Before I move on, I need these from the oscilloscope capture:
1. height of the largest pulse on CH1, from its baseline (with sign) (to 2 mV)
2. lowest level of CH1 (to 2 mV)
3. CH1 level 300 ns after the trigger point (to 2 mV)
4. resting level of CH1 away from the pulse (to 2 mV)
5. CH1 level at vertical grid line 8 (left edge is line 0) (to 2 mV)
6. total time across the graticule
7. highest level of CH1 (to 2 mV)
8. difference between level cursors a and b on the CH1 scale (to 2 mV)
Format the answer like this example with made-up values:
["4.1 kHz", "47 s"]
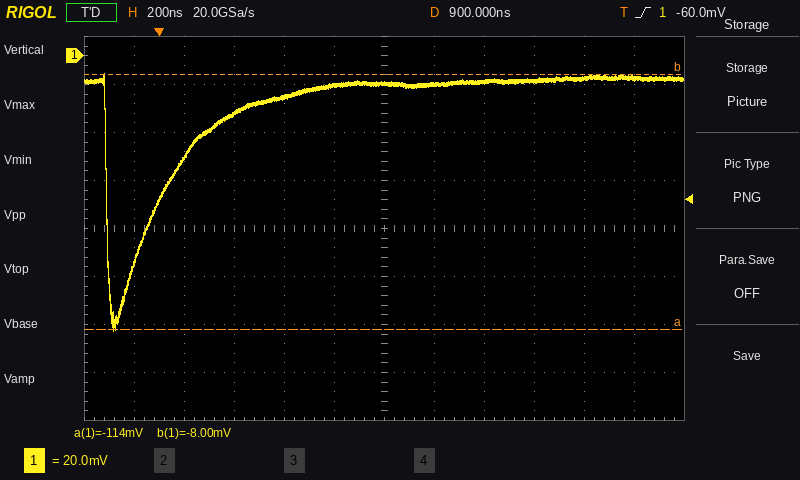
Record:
["-104 mV", "-114 mV", "-24 mV", "-10 mV", "-10 mV", "2.4 µs", "-8 mV", "106 mV"]
